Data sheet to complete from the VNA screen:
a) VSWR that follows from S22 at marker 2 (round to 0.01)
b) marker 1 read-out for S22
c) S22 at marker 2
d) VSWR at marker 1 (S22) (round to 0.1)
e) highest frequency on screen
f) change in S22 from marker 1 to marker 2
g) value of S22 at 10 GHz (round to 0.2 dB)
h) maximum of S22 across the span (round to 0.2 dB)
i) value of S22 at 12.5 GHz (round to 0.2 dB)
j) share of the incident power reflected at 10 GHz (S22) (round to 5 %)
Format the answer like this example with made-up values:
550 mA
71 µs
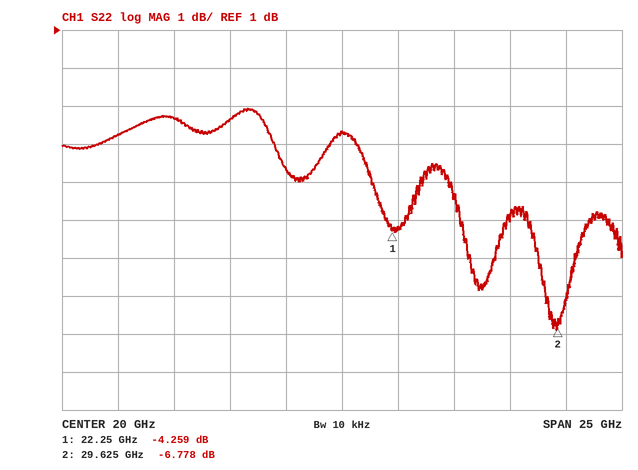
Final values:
2.69
-4.259 dB
-6.778 dB
4.2
32.5 GHz
-2.519 dB
-1.8 dB
-1.0 dB
-1.4 dB
65 %
